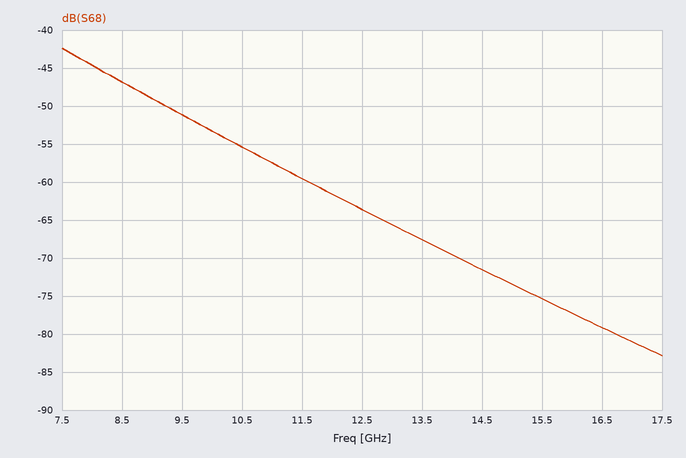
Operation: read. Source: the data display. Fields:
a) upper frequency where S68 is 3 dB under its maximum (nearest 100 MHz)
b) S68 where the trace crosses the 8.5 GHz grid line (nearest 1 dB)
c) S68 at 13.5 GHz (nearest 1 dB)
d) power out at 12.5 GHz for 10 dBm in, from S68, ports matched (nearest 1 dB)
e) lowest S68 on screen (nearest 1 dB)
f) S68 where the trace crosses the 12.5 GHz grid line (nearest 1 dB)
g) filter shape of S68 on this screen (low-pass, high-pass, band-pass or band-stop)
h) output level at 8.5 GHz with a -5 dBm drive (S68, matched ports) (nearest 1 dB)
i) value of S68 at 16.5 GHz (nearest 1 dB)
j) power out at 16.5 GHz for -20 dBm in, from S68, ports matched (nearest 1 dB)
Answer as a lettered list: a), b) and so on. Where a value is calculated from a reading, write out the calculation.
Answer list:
a) 8.2 GHz
b) -47 dB
c) -68 dB
d) 10 dBm + (-64 dB) = -54 dBm
e) -83 dB
f) -64 dB
g) low-pass
h) -5 dBm + (-47 dB) = -52 dBm
i) -79 dB
j) -20 dBm + (-79 dB) = -99 dBm
